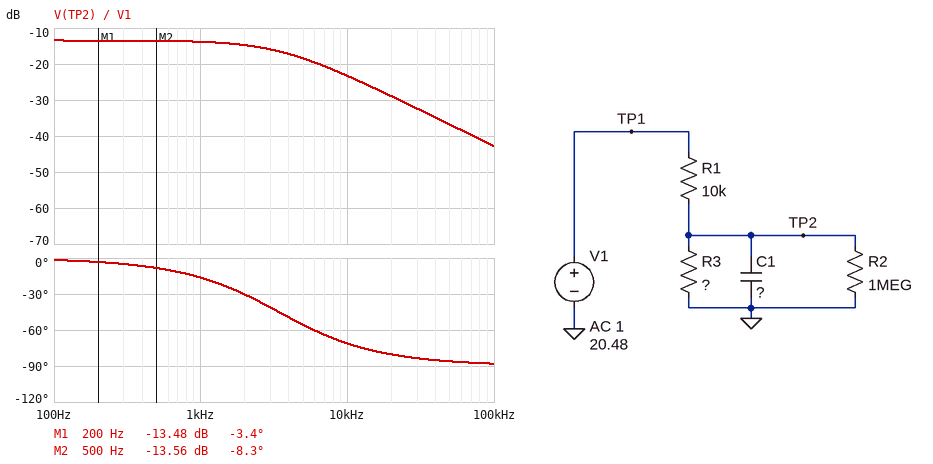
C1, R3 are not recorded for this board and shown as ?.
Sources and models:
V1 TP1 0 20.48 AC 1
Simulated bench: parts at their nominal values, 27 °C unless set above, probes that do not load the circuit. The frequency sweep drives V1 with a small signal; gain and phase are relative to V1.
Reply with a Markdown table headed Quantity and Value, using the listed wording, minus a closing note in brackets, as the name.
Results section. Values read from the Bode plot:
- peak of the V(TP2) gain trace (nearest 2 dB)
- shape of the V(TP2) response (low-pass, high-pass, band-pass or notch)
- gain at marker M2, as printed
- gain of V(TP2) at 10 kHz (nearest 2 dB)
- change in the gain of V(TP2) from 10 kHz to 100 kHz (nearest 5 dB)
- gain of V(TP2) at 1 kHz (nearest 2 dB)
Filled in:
| Quantity | Value |
|---|---|
| peak of the V(TP2) gain trace | -14 dB |
| shape of the V(TP2) response | low-pass |
| gain at marker M2, as printed | -13.56 dB |
| gain of V(TP2) at 10 kHz | -24 dB |
| change in the gain of V(TP2) from 10 kHz to 100 kHz | -20 dB |
| gain of V(TP2) at 1 kHz | -14 dB |
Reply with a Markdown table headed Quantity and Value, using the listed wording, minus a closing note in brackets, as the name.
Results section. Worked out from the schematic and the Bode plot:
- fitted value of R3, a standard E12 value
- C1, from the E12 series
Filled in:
| Quantity | Value |
|---|---|
| fitted value of R3, a standard E12 value | 2.7 kΩ |
| C1, from the E12 series | 22 nF |
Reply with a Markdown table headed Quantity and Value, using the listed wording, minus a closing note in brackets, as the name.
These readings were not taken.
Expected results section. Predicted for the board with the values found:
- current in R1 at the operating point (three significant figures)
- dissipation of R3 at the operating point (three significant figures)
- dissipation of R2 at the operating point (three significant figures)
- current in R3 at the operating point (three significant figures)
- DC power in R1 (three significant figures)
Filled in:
| Quantity | Value |
|---|---|
| current in R1 at the operating point | 1.61 mA |
| dissipation of R3 at the operating point | 6.99 mW |
| dissipation of R2 at the operating point | 18.9 µW |
| current in R3 at the operating point | 1.61 mA |
| DC power in R1 | 26.0 mW |
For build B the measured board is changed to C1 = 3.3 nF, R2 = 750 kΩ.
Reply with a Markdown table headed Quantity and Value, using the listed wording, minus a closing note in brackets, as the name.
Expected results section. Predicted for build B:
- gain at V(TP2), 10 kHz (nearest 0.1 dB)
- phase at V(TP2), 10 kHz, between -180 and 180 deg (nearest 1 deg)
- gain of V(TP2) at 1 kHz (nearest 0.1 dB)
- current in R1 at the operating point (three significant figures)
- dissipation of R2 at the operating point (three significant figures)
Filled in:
| Quantity | Value |
|---|---|
| gain at V(TP2), 10 kHz | -14.2 dB |
| phase at V(TP2), 10 kHz, between -180 and 180 deg | -24 deg |
| gain of V(TP2) at 1 kHz | -13.5 dB |
| current in R1 at the operating point | 1.61 mA |
| dissipation of R2 at the operating point | 25.1 µW |
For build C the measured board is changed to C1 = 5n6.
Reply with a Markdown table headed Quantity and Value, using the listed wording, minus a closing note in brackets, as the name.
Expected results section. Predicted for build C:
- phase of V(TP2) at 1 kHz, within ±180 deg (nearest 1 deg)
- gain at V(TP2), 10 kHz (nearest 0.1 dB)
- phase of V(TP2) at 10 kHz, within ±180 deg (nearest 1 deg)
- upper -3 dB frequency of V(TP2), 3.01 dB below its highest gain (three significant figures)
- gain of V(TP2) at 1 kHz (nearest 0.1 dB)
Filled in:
| Quantity | Value |
|---|---|
| phase of V(TP2) at 1 kHz, within ±180 deg | -4 deg |
| gain at V(TP2), 10 kHz | -15.4 dB |
| phase of V(TP2) at 10 kHz, within ±180 deg | -37 deg |
| upper -3 dB frequency of V(TP2), 3.01 dB below its highest gain | 13.4 kHz |
| gain of V(TP2) at 1 kHz | -13.5 dB |
